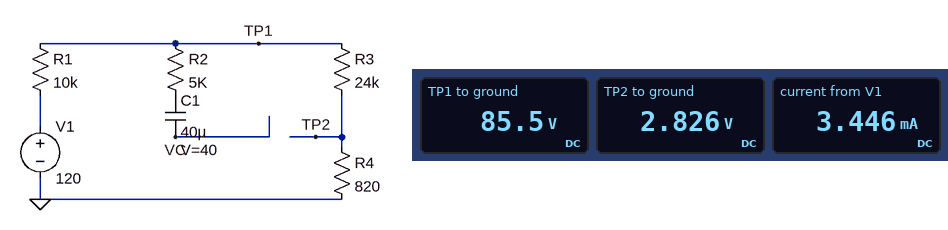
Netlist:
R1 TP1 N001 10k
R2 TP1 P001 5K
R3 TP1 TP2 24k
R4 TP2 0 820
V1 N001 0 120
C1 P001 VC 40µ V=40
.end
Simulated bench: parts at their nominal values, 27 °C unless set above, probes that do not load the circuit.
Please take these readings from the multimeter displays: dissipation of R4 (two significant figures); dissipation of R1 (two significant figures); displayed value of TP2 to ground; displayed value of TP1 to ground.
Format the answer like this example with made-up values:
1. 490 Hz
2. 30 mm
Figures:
1. 9.7 mW
2. 120 mW
3. 2.826 V
4. 85.5 V
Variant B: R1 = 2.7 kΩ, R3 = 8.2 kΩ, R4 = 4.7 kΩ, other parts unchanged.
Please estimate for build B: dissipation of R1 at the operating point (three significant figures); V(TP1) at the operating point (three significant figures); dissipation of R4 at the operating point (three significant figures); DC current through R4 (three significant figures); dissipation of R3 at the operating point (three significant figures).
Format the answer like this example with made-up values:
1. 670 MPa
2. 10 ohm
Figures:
1. 160 mW
2. 99.2 V
3. 278 mW
4. 7.69 mA
5. 485 mW
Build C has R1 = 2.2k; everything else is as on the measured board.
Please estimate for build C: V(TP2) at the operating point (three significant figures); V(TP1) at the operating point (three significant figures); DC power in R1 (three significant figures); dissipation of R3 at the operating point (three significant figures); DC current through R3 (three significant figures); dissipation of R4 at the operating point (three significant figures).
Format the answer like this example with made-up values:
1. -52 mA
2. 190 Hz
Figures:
1. 3.64 V
2. 110 V
3. 43.4 mW
4. 473 mW
5. 4.44 mA
6. 16.2 mW
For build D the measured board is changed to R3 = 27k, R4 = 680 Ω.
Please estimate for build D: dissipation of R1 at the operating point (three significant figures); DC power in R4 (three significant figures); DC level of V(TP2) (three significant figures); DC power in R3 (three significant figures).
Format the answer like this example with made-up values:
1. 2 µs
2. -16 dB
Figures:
1. 101 mW
2. 6.90 mW
3. 2.17 V
4. 274 mW
